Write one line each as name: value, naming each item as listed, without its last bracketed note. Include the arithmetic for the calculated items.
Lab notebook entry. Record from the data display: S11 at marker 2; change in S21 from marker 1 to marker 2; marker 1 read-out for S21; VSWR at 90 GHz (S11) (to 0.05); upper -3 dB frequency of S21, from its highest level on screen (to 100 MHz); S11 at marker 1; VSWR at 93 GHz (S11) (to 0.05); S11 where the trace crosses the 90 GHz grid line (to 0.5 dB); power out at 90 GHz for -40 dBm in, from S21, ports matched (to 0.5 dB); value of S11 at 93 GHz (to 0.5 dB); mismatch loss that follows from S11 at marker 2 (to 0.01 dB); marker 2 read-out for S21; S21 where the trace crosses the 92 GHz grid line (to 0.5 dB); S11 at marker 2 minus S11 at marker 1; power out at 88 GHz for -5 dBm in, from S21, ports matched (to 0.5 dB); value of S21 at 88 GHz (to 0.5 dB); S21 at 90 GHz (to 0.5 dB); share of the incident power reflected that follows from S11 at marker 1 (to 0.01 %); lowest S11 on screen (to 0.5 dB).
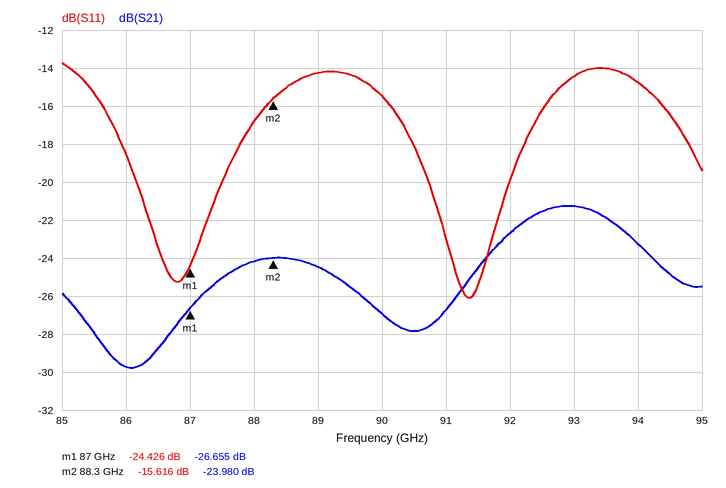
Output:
S11 at marker 2: -15.616 dB
change in S21 from marker 1 to marker 2: -23.98 − (-26.655) = 2.675 dB
marker 1 read-out for S21: -26.655 dB
VSWR at 90 GHz (S11): |Γ| = 10^(-15.5/20) = 0.1679; VSWR = (1 + 0.1679)/(1 − 0.1679) ≈ 1.40
upper -3 dB frequency of S21, from its highest level on screen: 94.3 GHz
S11 at marker 1: -24.426 dB
VSWR at 93 GHz (S11): |Γ| = 10^(-14.5/20) = 0.1884; VSWR = (1 + 0.1884)/(1 − 0.1884) ≈ 1.46, so 1.45 to the nearest 0.05
S11 where the trace crosses the 90 GHz grid line: -15.5 dB
power out at 90 GHz for -40 dBm in, from S21, ports matched: -40 dBm + (-27.0 dB) = -67.0 dBm
value of S11 at 93 GHz: -14.5 dB
mismatch loss that follows from S11 at marker 2: −10 log10(1 − 10^(-15.616/10)) ≈ 0.12 dB
marker 2 read-out for S21: -23.980 dB
S21 where the trace crosses the 92 GHz grid line: -22.5 dB
S11 at marker 2 minus S11 at marker 1: -15.616 − (-24.426) = 8.810 dB
power out at 88 GHz for -5 dBm in, from S21, ports matched: -5 dBm + (-24.0 dB) = -29.0 dBm
value of S21 at 88 GHz: -24.0 dB
S21 at 90 GHz: -27.0 dB
share of the incident power reflected that follows from S11 at marker 1: 10^(-24.426/10) ≈ 0.36 %
lowest S11 on screen: -26.0 dB
